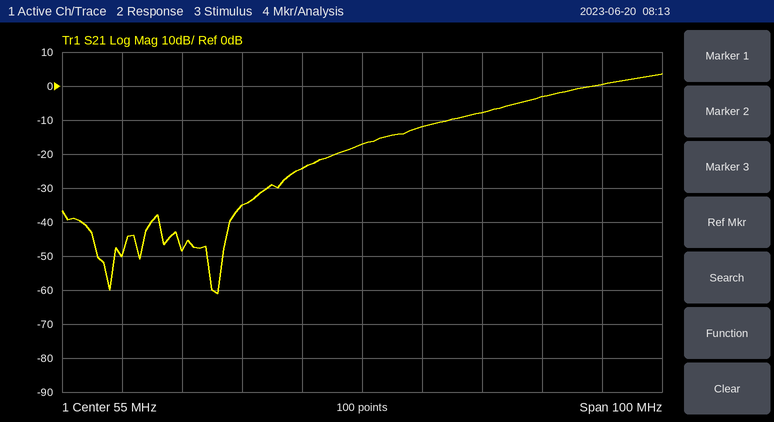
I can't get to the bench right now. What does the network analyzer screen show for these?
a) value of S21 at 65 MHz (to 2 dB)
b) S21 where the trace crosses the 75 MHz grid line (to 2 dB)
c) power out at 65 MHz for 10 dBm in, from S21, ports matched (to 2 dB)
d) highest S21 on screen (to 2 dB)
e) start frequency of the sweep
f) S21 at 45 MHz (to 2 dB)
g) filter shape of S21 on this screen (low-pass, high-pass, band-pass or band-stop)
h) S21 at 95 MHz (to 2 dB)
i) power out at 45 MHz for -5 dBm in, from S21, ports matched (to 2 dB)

-12 dB
-8 dB
-2 dBm
4 dB
5 MHz
-24 dB
high-pass
0 dB
-30 dBm
